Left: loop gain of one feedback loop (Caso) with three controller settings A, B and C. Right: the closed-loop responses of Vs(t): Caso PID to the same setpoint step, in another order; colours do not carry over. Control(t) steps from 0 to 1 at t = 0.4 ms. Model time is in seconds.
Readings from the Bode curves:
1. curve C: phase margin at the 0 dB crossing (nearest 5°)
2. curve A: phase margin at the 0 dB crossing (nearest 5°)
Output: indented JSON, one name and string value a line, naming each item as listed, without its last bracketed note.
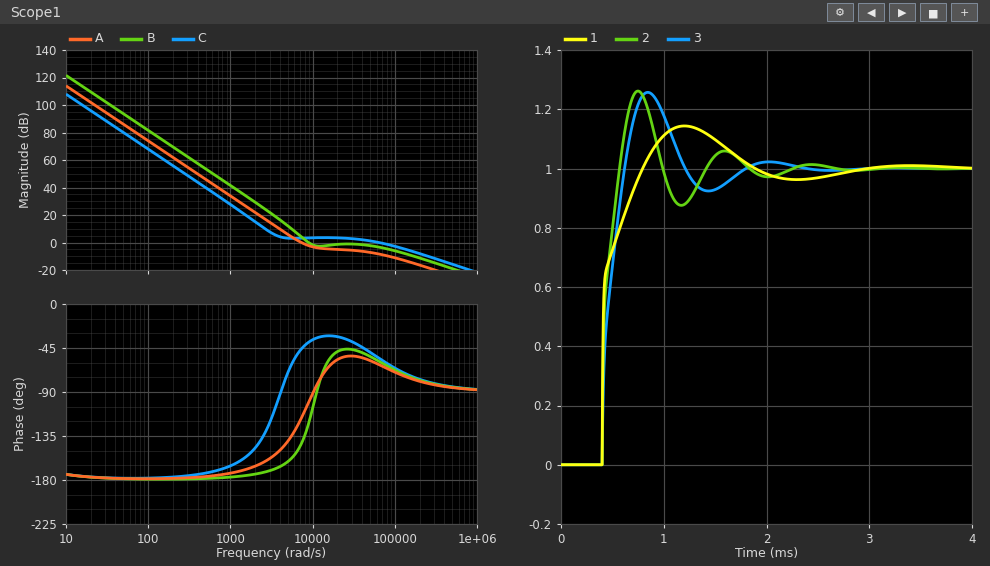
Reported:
{
  "curve C: phase margin at the 0 dB crossing": "125°",
  "curve A: phase margin at the 0 dB crossing": "65°"
}
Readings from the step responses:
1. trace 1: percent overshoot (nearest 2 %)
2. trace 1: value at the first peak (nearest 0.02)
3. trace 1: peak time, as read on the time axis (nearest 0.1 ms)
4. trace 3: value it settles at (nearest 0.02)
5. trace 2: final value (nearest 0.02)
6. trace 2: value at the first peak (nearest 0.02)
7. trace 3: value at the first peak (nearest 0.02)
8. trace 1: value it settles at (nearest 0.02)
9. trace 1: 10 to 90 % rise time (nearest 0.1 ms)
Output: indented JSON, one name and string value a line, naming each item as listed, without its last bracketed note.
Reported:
{
  "trace 1: percent overshoot": "14 %",
  "trace 1: value at the first peak": "1.14",
  "trace 1: peak time, as read on the time axis": "1.2 ms",
  "trace 3: value it settles at": "1.00",
  "trace 2: final value": "1.00",
  "trace 2: value at the first peak": "1.26",
  "trace 3: value at the first peak": "1.26",
  "trace 1: value it settles at": "1.00",
  "trace 1: 10 to 90 % rise time": "0.3 ms"
}
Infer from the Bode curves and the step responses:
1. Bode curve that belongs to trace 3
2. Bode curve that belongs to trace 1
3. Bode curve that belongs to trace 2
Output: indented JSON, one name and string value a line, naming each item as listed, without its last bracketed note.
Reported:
{
  "Bode curve that belongs to trace 3": "A",
  "Bode curve that belongs to trace 1": "C",
  "Bode curve that belongs to trace 2": "B"
}
